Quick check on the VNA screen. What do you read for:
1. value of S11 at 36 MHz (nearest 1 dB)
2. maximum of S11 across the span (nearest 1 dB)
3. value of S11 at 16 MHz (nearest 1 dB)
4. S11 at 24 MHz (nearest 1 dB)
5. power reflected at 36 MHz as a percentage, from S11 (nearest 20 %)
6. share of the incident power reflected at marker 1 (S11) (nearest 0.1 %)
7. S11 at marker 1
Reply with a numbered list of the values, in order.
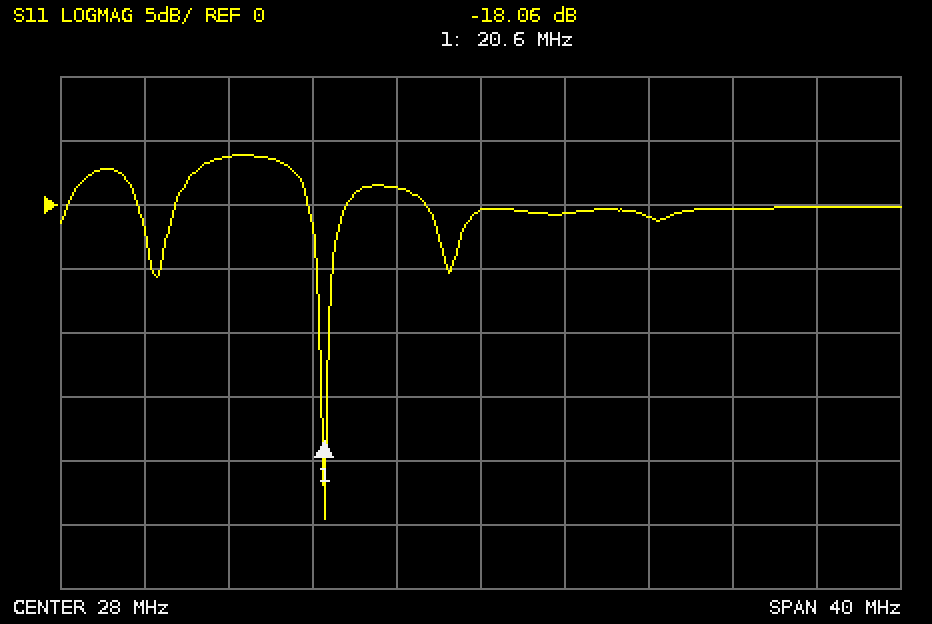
1. -1 dB
2. 4 dB
3. 4 dB
4. 1 dB
5. 80 %
6. 1.6 %
7. -18.06 dB
